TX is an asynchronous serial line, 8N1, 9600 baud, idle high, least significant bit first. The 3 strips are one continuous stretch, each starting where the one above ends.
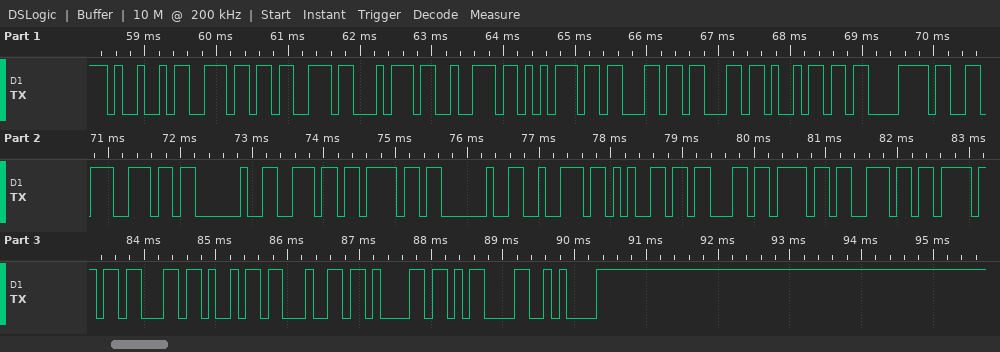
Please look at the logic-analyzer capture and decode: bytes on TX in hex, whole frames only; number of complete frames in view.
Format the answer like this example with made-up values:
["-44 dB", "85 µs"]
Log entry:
["49 6E 73 74 72 75 63 63 69 C3 B3 6E 20 6E 6F 20 72 65 63 6F 6E 6F 63 69 64 61 0D 0A", "28"]
